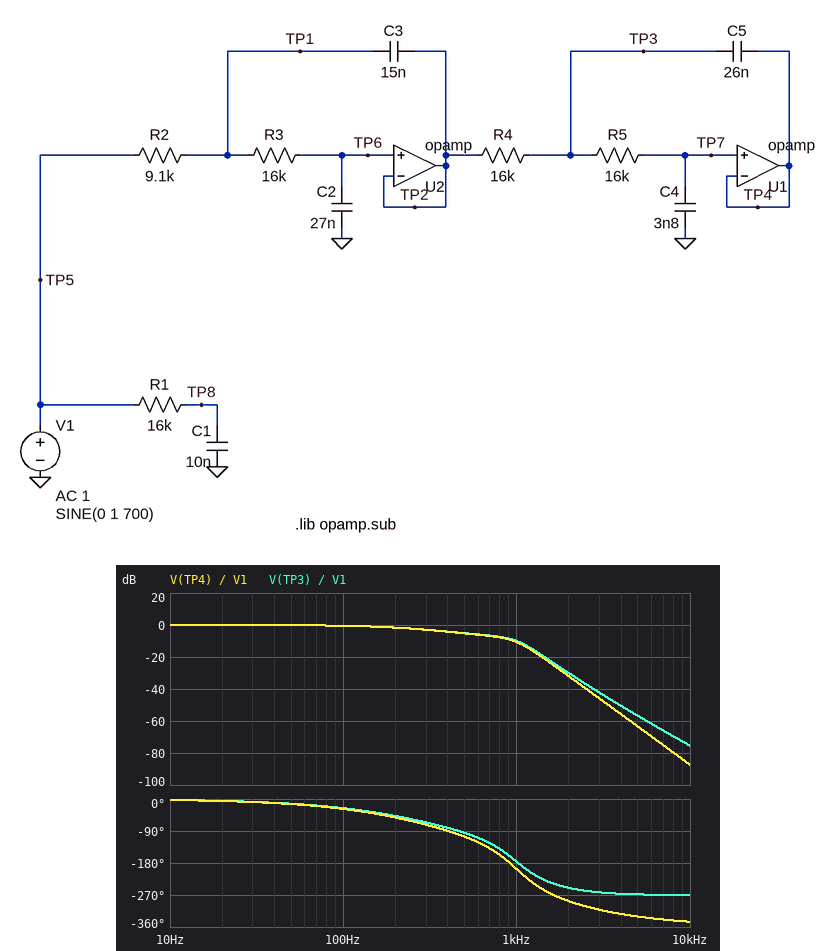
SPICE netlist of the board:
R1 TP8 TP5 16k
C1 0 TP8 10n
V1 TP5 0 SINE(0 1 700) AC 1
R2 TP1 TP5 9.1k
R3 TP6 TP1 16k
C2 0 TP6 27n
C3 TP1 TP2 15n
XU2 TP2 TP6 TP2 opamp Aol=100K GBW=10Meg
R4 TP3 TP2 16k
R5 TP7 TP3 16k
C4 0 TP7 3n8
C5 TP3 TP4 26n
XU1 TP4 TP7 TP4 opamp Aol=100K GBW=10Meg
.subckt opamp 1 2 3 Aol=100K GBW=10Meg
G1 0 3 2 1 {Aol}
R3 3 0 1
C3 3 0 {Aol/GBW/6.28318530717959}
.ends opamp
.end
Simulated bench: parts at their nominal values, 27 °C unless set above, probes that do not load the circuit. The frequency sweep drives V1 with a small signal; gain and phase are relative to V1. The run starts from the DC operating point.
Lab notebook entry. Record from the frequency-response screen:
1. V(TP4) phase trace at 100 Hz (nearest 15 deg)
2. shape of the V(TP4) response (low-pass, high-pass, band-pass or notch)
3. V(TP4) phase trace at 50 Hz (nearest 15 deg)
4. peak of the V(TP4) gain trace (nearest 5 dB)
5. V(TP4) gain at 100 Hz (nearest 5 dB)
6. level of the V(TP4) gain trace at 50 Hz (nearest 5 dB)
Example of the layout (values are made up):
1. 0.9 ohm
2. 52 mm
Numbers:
1. -30 deg
2. low-pass
3. -15 deg
4. 0 dB
5. 0 dB
6. 0 dB
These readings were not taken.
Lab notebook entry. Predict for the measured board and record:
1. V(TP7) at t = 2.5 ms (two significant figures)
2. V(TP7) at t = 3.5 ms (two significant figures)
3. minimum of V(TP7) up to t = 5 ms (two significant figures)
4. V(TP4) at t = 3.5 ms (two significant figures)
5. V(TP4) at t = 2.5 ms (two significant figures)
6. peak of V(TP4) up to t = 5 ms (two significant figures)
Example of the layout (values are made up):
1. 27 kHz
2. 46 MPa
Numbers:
1. 350 mV
2. 180 mV
3. -450 mV
4. 180 mV
5. 350 mV
6. 520 mV
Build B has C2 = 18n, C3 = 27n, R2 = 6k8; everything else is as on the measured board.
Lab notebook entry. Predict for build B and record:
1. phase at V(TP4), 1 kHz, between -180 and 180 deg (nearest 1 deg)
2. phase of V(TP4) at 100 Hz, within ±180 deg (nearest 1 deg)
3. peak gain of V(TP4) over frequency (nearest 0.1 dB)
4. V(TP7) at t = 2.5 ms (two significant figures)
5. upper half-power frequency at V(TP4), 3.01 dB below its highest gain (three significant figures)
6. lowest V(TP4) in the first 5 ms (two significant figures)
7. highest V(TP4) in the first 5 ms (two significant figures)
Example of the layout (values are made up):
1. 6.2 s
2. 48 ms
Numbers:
1. 157 deg
2. -19 deg
3. 0 dB
4. 550 mV
5. 759 Hz
6. -750 mV
7. 750 mV
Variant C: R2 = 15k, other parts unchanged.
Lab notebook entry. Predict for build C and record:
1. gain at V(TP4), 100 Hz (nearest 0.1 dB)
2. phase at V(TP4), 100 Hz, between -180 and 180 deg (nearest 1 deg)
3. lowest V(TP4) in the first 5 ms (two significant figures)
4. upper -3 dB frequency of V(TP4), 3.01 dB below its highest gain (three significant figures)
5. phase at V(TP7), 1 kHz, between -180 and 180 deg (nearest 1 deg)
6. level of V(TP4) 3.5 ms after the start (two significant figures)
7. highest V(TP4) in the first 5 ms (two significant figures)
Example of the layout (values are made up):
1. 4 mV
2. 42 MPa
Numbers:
1. -0.7 dB
2. -33 deg
3. -360 mV
4. 237 Hz
5. 152 deg
6. 78 mV
7. 440 mV
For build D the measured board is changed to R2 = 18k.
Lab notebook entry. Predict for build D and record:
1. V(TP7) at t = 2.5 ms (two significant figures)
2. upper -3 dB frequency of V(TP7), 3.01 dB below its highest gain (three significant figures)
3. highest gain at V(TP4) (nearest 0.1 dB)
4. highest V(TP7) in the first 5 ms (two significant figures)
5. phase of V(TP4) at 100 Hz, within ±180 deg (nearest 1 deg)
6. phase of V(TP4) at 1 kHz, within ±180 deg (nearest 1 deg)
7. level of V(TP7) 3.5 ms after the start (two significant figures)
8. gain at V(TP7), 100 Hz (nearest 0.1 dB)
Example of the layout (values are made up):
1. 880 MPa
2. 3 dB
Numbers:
1. 300 mV
2. 213 Hz
3. 0 dB
4. 410 mV
5. -36 deg
6. 148 deg
7. 51 mV
8. -0.9 dB
